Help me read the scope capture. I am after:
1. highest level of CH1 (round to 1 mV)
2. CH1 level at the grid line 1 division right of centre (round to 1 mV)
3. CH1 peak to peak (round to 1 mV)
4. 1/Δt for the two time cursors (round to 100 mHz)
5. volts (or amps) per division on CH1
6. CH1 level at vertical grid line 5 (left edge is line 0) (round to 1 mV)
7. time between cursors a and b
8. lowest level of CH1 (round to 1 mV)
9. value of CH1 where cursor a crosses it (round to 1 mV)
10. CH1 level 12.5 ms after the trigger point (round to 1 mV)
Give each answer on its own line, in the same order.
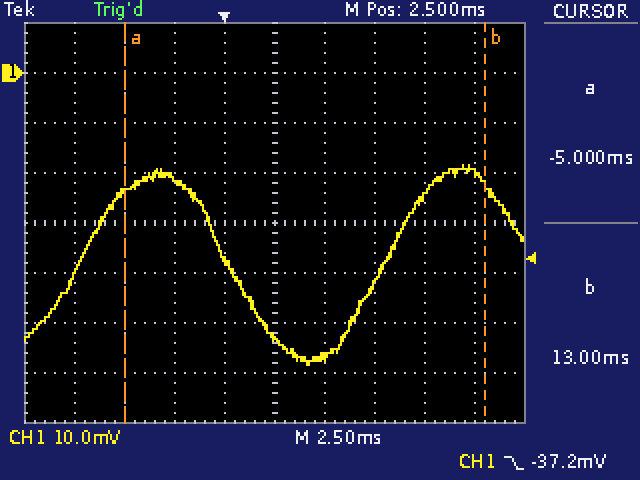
-18 mV
-57 mV
40 mV
55.6 Hz
10 mV
-53 mV
18.00 ms
-58 mV
-24 mV
-20 mV
